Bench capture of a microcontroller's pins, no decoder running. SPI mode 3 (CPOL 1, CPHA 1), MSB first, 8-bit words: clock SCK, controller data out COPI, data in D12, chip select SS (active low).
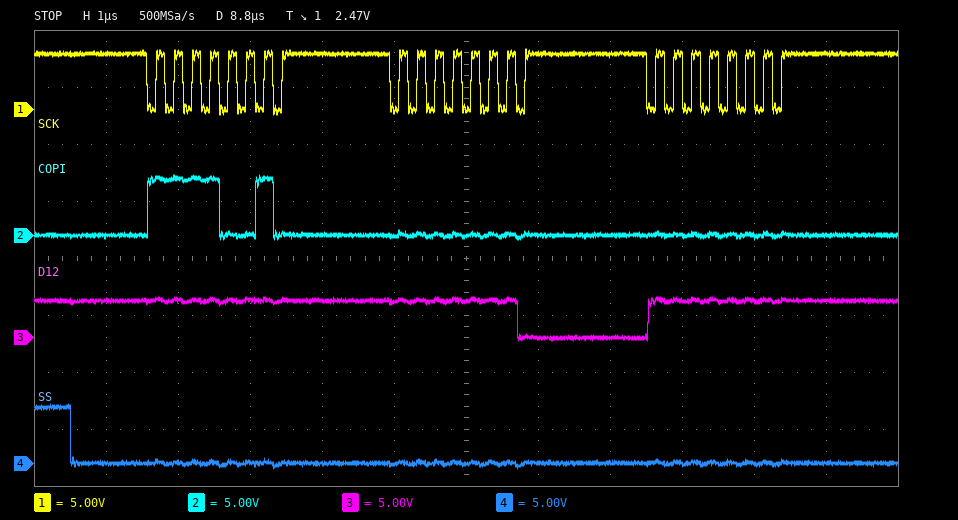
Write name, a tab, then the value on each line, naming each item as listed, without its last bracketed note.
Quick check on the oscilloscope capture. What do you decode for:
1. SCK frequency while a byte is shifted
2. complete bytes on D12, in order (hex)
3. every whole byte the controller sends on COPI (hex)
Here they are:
SCK frequency while a byte is shifted	4 MHz
complete bytes on D12, in order	0xFF 0xFE 0xFF
every whole byte the controller sends on COPI	0xF2 0x00 0x00
